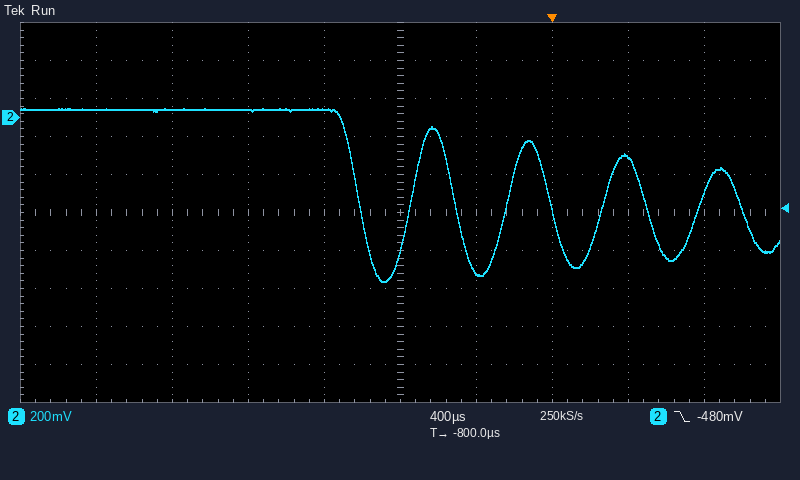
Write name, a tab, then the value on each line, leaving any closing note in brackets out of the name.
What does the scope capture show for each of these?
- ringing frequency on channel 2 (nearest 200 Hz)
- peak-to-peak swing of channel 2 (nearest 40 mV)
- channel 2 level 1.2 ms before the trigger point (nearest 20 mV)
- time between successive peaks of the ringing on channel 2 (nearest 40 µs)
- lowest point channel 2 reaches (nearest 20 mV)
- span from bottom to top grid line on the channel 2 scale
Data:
ringing frequency on channel 2	2.0 kHz
peak-to-peak swing of channel 2	920 mV
channel 2 level 1.2 ms before the trigger point	40 mV
time between successive peaks of the ringing on channel 2	520 µs
lowest point channel 2 reaches	-860 mV
span from bottom to top grid line on the channel 2 scale	2 V
